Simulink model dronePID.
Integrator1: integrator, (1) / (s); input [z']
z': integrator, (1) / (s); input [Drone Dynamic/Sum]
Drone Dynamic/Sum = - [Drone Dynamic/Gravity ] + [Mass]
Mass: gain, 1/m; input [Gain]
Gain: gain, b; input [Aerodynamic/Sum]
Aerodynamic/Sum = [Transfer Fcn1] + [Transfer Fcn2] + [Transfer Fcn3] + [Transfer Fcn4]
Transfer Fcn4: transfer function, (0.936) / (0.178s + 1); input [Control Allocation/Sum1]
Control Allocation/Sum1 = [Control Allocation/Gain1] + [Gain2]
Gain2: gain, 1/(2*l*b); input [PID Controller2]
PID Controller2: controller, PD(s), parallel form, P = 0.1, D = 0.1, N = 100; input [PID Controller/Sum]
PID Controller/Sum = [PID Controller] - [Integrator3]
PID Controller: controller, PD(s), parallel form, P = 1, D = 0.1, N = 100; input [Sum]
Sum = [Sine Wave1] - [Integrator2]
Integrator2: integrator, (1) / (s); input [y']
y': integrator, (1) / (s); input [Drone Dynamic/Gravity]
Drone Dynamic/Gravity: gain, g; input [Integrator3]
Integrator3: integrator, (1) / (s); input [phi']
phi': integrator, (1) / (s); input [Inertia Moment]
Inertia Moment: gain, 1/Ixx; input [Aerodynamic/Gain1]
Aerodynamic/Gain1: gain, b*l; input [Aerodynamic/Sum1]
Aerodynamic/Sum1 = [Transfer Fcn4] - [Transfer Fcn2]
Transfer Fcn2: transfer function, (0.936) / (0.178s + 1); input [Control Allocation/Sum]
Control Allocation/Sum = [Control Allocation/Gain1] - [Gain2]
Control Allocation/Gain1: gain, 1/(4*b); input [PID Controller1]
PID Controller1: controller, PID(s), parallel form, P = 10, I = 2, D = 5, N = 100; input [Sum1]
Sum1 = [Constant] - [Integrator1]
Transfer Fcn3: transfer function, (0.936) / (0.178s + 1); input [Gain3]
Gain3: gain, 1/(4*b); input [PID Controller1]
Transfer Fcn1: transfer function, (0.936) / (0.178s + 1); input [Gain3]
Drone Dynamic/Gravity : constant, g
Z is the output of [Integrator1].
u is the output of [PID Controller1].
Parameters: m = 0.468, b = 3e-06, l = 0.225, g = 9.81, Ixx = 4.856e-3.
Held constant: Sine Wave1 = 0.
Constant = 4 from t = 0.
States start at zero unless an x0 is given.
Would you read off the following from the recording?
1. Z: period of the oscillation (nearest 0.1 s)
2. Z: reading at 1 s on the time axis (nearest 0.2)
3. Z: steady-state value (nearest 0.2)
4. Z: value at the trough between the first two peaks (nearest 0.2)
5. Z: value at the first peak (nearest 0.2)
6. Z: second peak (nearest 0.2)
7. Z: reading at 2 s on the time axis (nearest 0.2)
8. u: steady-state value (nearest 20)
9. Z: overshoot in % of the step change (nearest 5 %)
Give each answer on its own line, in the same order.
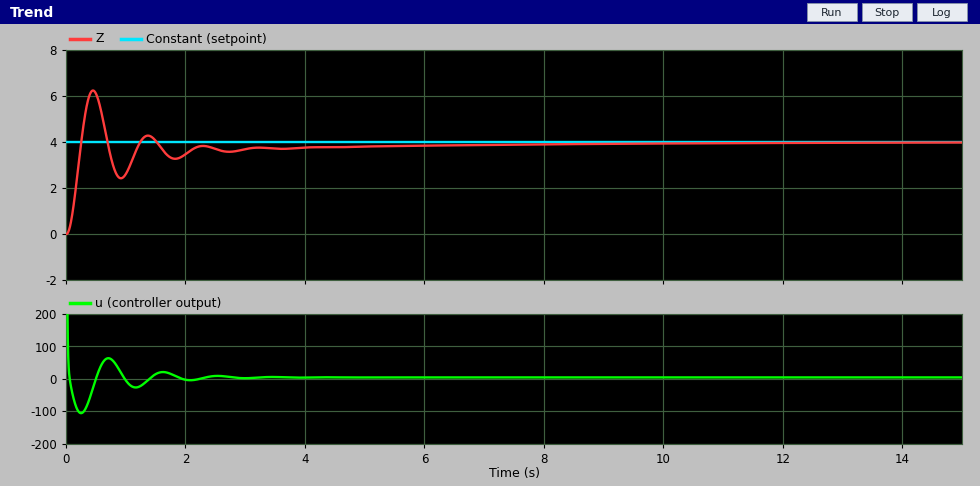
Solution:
0.9 s
2.6
4.0
2.4
6.2
4.2
3.4
0
55 %
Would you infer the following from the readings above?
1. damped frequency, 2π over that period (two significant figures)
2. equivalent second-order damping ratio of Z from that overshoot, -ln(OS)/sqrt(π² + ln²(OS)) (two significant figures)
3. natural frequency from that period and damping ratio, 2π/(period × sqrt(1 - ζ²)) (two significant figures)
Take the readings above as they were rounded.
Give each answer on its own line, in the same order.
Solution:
7.0 rad/s
0.19
7.1 rad/s
